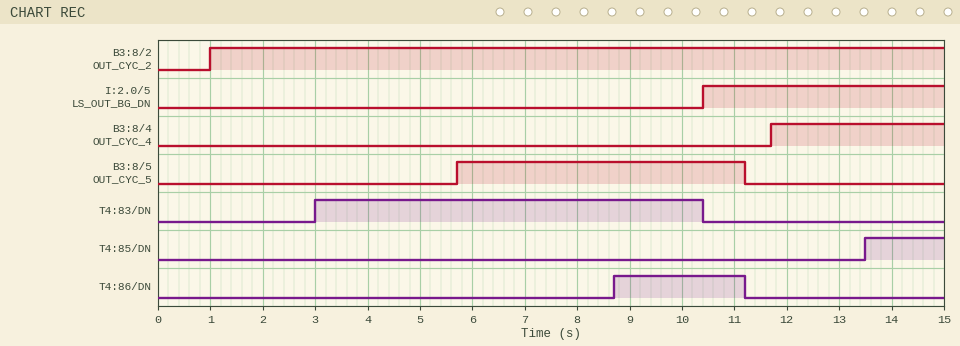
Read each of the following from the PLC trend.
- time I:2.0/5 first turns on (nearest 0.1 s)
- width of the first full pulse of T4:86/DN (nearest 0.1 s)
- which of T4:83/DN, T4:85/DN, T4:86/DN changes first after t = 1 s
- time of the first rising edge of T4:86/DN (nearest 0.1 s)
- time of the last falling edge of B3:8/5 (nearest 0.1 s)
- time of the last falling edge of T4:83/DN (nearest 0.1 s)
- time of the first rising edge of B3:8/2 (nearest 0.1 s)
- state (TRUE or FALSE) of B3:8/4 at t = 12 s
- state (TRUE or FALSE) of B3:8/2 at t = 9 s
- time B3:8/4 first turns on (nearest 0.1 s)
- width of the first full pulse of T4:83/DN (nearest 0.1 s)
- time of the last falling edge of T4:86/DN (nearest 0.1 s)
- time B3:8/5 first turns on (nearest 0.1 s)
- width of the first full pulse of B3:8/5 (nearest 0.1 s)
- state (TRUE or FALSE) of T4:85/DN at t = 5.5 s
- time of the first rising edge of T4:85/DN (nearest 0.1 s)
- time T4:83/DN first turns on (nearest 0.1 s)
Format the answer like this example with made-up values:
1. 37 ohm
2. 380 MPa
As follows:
1. 10.4 s
2. 2.5 s
3. T4:83/DN
4. 8.7 s
5. 11.2 s
6. 10.4 s
7. 1.0 s
8. TRUE
9. TRUE
10. 11.7 s
11. 7.4 s
12. 11.2 s
13. 5.7 s
14. 5.5 s
15. FALSE
16. 13.5 s
17. 3.0 s
